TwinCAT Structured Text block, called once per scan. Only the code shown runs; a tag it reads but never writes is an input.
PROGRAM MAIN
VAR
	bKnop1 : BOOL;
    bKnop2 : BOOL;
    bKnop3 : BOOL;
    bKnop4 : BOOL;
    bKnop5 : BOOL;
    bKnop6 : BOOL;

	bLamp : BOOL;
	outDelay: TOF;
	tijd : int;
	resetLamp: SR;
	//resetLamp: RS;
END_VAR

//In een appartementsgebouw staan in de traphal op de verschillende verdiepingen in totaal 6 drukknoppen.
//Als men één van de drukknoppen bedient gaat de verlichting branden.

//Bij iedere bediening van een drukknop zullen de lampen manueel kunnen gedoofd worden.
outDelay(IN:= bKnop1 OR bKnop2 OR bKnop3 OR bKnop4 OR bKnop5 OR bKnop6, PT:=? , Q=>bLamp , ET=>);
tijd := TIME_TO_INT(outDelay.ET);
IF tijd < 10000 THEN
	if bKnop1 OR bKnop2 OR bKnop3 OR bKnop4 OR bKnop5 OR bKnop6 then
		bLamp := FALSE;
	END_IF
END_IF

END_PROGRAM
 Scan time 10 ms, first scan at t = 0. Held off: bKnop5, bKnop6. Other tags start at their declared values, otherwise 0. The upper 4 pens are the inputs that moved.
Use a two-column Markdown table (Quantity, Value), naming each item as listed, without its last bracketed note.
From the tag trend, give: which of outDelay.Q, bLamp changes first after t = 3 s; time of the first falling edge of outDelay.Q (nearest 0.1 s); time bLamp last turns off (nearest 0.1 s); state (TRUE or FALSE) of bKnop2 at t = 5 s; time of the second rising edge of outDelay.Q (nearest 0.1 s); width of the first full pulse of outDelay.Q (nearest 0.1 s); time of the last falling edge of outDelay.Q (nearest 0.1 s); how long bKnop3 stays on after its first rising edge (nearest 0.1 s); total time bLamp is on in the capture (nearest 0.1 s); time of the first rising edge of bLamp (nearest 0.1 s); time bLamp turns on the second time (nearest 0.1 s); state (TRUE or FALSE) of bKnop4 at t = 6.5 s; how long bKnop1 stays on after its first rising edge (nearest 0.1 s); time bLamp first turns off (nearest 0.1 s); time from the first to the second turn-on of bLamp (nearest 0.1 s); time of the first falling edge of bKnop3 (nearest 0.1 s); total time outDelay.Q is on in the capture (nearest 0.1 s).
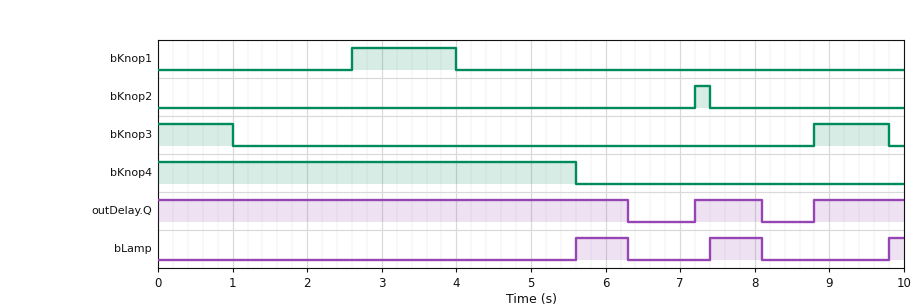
| Quantity | Value |
|---|---|
| which of outDelay.Q, bLamp changes first after t = 3 s | bLamp |
| time of the first falling edge of outDelay.Q | 6.3 s |
| time bLamp last turns off | 8.1 s |
| state (TRUE or FALSE) of bKnop2 at t = 5 s | FALSE |
| time of the second rising edge of outDelay.Q | 8.8 s |
| width of the first full pulse of outDelay.Q | 0.9 s |
| time of the last falling edge of outDelay.Q | 8.1 s |
| how long bKnop3 stays on after its first rising edge | 1.0 s |
| total time bLamp is on in the capture | 1.6 s |
| time of the first rising edge of bLamp | 5.6 s |
| time bLamp turns on the second time | 7.4 s |
| state (TRUE or FALSE) of bKnop4 at t = 6.5 s | FALSE |
| how long bKnop1 stays on after its first rising edge | 1.4 s |
| time bLamp first turns off | 6.3 s |
| time from the first to the second turn-on of bLamp | 1.8 s |
| time of the first falling edge of bKnop3 | 1.0 s |
| total time outDelay.Q is on in the capture | 8.4 s |
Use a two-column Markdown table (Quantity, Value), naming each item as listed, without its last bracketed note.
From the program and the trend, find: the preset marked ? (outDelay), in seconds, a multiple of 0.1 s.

| Quantity | Value |
|---|---|
| the preset marked ? (outDelay), in seconds, a multiple of 0.1 s | 0.7 s |
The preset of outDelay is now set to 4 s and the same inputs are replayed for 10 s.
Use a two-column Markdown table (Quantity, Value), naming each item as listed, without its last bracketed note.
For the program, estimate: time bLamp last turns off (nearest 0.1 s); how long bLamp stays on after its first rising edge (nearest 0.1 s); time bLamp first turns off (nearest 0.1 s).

| Quantity | Value |
|---|---|
| time bLamp last turns off | 8.8 s |
| how long bLamp stays on after its first rising edge | 1.6 s |
| time bLamp first turns off | 7.2 s |
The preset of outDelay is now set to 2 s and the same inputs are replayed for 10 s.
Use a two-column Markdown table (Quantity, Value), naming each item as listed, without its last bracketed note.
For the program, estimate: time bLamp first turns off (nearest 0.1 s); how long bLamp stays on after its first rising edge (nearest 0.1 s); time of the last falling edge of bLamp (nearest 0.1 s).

| Quantity | Value |
|---|---|
| time bLamp first turns off | 7.2 s |
| how long bLamp stays on after its first rising edge | 1.6 s |
| time of the last falling edge of bLamp | 8.8 s |
